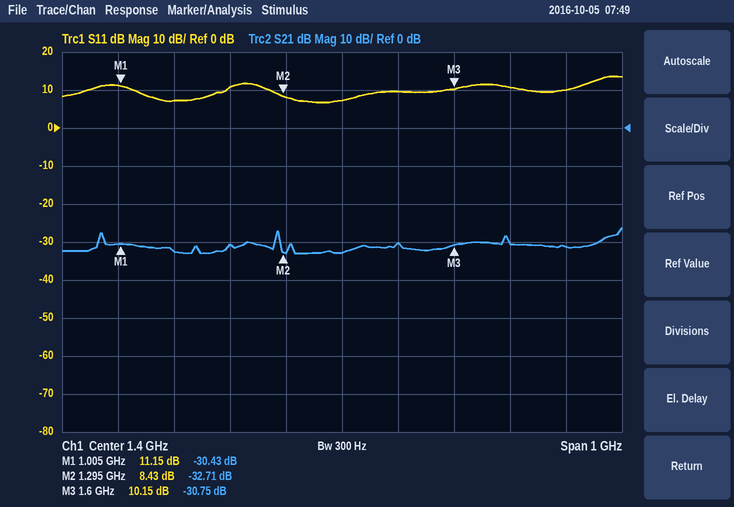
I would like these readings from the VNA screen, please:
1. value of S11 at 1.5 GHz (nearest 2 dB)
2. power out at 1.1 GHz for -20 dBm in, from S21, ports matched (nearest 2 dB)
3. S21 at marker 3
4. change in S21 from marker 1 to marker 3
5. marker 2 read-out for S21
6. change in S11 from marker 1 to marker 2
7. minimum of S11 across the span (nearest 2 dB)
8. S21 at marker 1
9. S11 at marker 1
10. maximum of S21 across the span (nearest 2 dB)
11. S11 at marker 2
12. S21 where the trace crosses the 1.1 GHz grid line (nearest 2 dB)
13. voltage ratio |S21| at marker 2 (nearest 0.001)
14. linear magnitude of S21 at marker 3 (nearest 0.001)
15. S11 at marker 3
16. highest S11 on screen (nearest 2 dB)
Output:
10 dB
-52 dBm
-30.75 dB
-0.32 dB
-32.71 dB
-2.72 dB
6 dB
-30.43 dB
11.15 dB
-26 dB
8.43 dB
-32 dB
0.023
0.029
10.15 dB
14 dB
